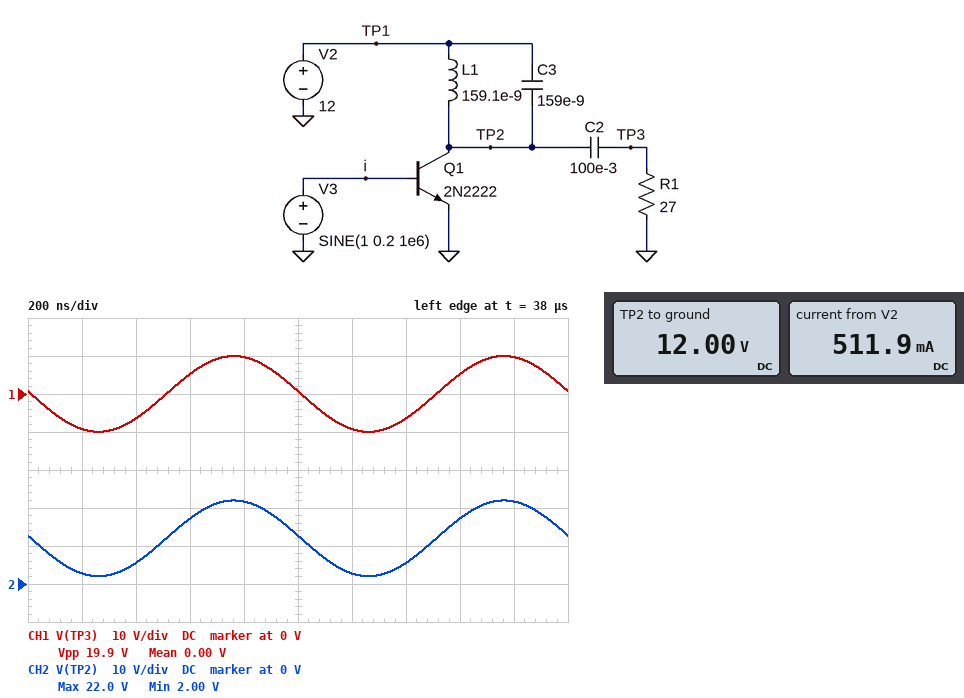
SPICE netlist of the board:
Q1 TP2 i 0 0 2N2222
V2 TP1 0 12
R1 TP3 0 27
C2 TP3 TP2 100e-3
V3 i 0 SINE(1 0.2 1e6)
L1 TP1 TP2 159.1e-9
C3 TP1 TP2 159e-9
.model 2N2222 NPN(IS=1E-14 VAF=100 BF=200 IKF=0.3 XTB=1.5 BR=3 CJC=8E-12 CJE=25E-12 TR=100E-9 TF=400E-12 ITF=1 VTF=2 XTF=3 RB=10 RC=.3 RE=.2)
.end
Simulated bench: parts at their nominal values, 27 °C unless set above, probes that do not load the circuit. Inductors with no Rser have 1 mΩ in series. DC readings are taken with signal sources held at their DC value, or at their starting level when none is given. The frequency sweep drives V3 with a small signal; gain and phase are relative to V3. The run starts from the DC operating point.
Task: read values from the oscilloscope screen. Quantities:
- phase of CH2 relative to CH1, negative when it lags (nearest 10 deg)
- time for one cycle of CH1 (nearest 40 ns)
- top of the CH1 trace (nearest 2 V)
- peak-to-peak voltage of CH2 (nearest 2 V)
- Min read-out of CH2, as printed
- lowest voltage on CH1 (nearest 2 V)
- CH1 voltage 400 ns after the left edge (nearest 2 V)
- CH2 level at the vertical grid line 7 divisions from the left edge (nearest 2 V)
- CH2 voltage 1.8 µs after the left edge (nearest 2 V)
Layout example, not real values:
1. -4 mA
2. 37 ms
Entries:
1. 0 deg
2. 1.00 µs
3. 10 V
4. 20 V
5. 2.00 V
6. -10 V
7. -6 V
8. 6 V
9. 22 V
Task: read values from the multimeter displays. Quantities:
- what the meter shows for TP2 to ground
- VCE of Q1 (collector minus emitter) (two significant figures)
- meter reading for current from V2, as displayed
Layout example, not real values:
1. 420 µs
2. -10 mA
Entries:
1. 12.00 V
2. 12 V
3. 511.9 mA
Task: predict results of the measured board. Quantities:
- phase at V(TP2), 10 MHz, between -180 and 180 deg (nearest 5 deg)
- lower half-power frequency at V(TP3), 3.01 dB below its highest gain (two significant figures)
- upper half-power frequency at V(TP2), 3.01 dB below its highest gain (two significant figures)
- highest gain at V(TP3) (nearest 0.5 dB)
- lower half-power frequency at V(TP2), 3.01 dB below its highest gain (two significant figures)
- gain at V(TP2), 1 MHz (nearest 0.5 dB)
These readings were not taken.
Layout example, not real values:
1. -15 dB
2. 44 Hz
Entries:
1. 60 deg
2. 980 kHz
3. 1.0 MHz
4. 34.5 dB
5. 980 kHz
6. 34.5 dB
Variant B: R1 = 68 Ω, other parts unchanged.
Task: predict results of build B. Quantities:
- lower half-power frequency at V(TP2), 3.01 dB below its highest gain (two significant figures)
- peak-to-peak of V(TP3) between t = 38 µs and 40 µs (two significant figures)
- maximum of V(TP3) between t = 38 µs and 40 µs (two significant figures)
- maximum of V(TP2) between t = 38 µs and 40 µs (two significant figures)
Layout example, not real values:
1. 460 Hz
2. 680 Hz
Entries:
1. 990 kHz
2. 28 V
3. 14 V
4. 26 V
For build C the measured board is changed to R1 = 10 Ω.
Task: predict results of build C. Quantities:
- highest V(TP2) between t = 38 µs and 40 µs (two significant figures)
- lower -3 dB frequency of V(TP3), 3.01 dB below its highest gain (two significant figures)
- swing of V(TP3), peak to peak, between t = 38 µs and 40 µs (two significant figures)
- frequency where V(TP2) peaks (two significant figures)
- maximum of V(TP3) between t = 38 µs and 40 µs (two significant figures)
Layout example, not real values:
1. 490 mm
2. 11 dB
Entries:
1. 16 V
2. 950 kHz
3. 7.9 V
4. 1.0 MHz
5. 4.0 V
